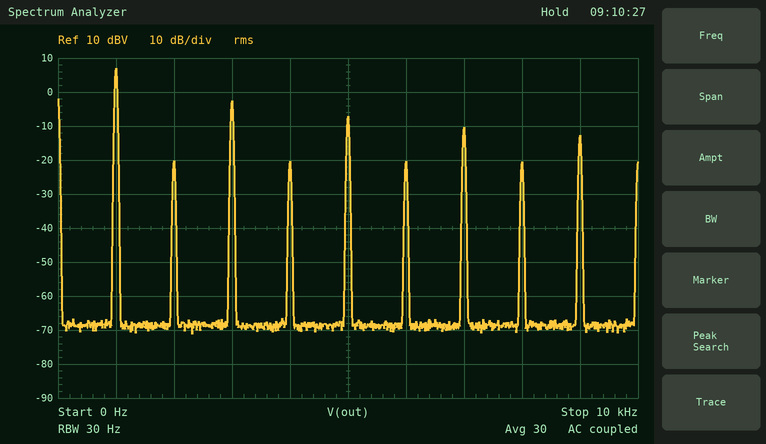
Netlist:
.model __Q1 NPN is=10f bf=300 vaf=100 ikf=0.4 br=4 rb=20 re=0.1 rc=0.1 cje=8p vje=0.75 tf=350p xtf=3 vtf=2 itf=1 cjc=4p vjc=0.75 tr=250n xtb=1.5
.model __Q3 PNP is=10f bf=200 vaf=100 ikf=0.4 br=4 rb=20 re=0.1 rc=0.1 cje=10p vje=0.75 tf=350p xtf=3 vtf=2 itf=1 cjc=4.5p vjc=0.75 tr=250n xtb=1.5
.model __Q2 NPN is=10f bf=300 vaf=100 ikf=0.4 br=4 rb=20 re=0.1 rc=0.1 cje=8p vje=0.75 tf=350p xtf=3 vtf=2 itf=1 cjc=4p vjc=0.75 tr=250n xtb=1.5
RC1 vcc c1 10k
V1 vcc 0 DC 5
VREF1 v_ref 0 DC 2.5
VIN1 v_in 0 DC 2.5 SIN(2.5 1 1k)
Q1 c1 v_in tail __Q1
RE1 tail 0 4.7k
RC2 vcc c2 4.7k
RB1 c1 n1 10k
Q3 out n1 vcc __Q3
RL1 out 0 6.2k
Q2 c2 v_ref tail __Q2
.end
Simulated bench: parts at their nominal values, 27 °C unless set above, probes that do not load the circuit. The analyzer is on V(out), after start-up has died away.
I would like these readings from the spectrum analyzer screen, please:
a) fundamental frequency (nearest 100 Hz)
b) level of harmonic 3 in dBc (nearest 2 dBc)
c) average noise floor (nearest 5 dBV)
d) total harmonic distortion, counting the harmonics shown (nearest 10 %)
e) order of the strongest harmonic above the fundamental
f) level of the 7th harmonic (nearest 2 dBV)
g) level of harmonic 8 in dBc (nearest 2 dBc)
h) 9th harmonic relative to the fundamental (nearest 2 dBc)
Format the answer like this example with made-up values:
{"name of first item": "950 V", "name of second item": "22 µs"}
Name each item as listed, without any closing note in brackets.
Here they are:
{"fundamental frequency": "1.0 kHz", "level of harmonic 3 in dBc": "-10 dBc", "average noise floor": "-70 dBV", "total harmonic distortion, counting the harmonics shown": "40 %", "order of the strongest harmonic above the fundamental": "3", "level of the 7th harmonic": "-10 dBV", "level of harmonic 8 in dBc": "-28 dBc", "9th harmonic relative to the fundamental": "-20 dBc"}
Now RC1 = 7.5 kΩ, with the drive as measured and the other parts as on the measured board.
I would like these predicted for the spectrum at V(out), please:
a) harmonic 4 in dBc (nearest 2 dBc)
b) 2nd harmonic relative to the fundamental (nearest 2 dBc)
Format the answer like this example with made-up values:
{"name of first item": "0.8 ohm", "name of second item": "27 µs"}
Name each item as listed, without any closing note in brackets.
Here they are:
{"harmonic 4 in dBc": "-30 dBc", "2nd harmonic relative to the fundamental": "-30 dBc"}
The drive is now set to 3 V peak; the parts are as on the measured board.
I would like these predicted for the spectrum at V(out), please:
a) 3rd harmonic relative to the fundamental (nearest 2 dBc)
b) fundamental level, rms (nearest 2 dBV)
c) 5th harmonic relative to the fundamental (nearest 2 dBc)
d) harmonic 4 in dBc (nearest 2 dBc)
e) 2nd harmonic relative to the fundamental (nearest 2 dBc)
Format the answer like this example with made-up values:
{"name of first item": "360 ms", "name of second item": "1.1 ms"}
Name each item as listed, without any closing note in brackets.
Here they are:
{"3rd harmonic relative to the fundamental": "2 dBc", "fundamental level, rms": "0 dBV", "5th harmonic relative to the fundamental": "-12 dBc", "harmonic 4 in dBc": "-8 dBc", "2nd harmonic relative to the fundamental": "0 dBc"}
